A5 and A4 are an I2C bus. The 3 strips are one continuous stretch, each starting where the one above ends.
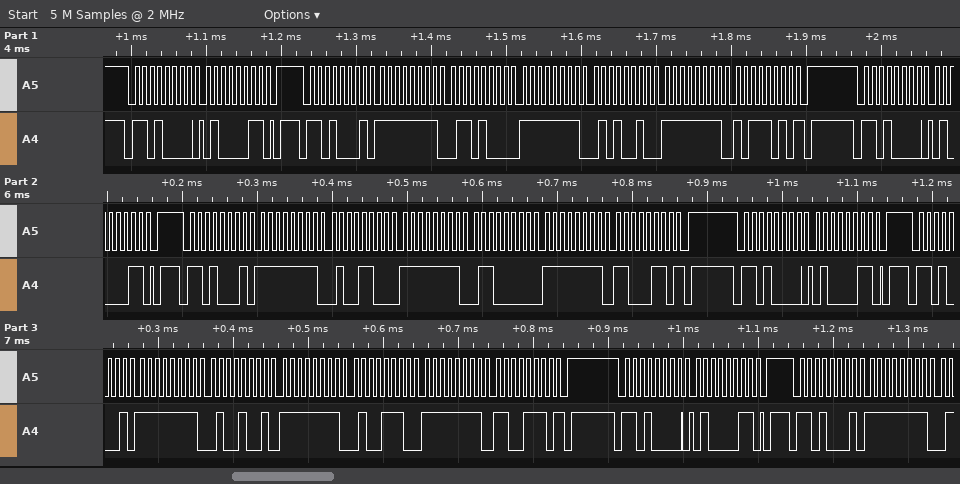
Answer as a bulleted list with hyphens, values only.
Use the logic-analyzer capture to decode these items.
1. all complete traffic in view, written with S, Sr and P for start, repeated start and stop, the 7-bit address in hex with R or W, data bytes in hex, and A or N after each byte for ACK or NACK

- S 68W A 43 A P S 68R A FF A 68 A FF A 52 A FF A BA N P S 68W A 43 A P S 68R A FF A 4C A FF A 60 A FF A C6 N P S 68W A 43 A P S 68R A FF A 49 A FF A 4E A FF A CE N P S 68W A 43 A P S 68R A FF A
